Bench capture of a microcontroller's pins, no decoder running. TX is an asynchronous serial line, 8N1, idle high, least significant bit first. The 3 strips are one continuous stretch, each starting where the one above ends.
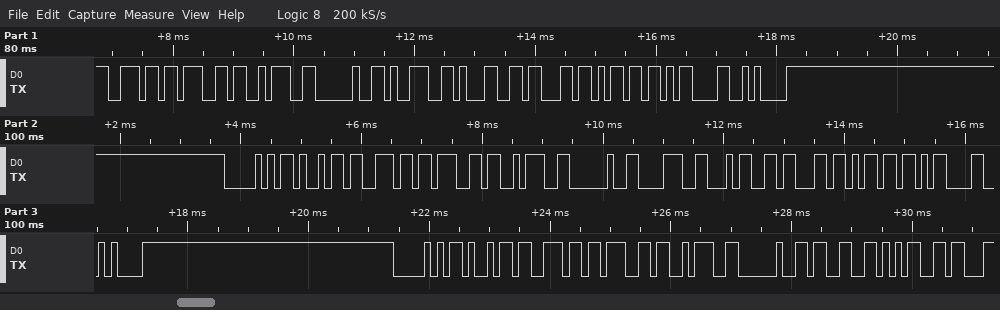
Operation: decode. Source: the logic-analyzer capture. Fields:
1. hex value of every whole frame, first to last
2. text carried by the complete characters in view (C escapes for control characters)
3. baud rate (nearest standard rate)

6E 67 3A 20 39 31 63 6D 0D 0A 50 69 6E 67 3A 20 38 34 63 6D 0D 0A 50 69 6E 67 3A 20 33 35
"ng: 91cm\r\nPing: 84cm\r\nPing: 35"
9600 baud
